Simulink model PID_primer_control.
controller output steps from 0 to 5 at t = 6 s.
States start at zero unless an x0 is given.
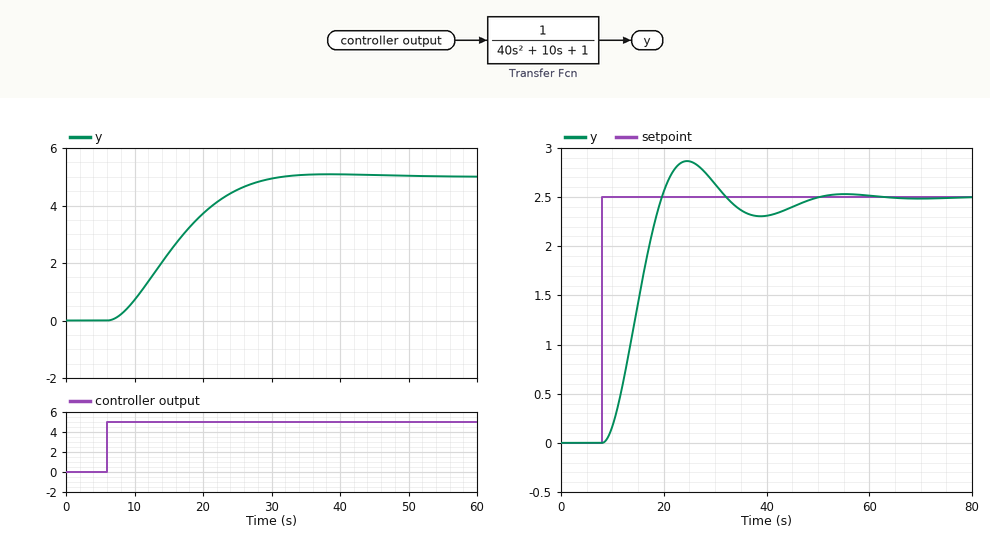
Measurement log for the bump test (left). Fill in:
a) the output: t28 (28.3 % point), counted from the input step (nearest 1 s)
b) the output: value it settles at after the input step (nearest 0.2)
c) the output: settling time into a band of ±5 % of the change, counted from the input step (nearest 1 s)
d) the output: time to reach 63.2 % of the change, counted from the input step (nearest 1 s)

6 s
5.0
21 s
12 s
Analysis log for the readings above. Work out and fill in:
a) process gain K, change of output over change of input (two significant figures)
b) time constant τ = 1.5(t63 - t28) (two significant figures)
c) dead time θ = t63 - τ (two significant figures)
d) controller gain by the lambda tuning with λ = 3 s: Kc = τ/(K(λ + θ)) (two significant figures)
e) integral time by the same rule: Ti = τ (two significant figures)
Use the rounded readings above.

1.0
9.0 s
3.0 s
1.5
9.0 s
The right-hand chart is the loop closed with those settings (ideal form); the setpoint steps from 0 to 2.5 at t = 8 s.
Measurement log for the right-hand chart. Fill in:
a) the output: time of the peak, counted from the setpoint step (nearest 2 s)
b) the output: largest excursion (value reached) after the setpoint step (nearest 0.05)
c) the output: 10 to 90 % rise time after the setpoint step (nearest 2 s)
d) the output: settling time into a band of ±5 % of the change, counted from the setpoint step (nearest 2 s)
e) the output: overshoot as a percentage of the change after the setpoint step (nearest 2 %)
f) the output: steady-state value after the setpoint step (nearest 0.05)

16 s
2.85
8 s
36 s
14 %
2.50
